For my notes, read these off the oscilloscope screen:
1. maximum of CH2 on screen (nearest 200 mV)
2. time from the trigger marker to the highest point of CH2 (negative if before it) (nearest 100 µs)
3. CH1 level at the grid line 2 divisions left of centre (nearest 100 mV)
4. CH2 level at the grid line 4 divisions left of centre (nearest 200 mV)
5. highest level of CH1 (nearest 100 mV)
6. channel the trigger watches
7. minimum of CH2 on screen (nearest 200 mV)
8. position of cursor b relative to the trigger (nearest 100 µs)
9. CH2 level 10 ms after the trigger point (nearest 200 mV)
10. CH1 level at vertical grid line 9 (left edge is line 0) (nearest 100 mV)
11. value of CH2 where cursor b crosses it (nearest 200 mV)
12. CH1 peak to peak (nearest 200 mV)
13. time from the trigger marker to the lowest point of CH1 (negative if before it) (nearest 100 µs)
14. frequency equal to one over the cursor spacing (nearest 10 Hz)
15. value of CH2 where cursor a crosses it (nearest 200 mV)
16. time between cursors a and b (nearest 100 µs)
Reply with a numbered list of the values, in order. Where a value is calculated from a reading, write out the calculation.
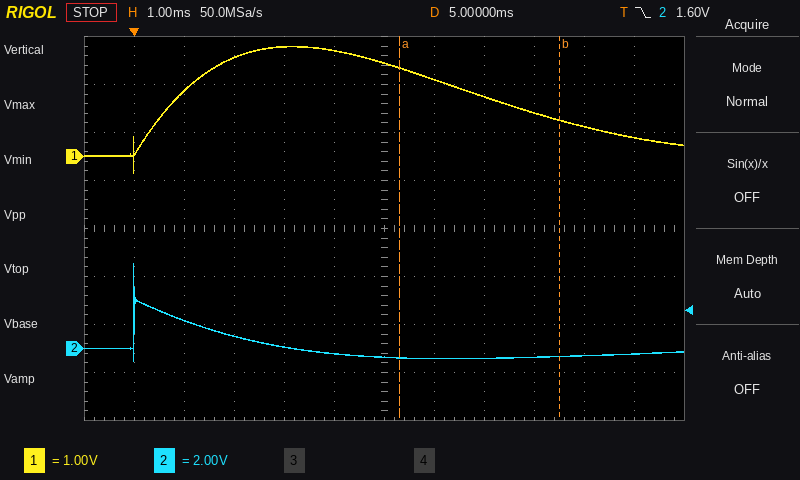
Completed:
1. 3.6 V
2. 0.0 ms
3. 2.3 V
4. 1.2 V
5. 2.3 V
6. CH2
7. -600 mV
8. +8.5 ms
9. -200 mV
10. 900 mV
11. -400 mV
12. 2.6 V
13. 0.0 ms
14. 1 / 3.2 ms ≈ 310 Hz
15. -400 mV
16. 3.2 ms
